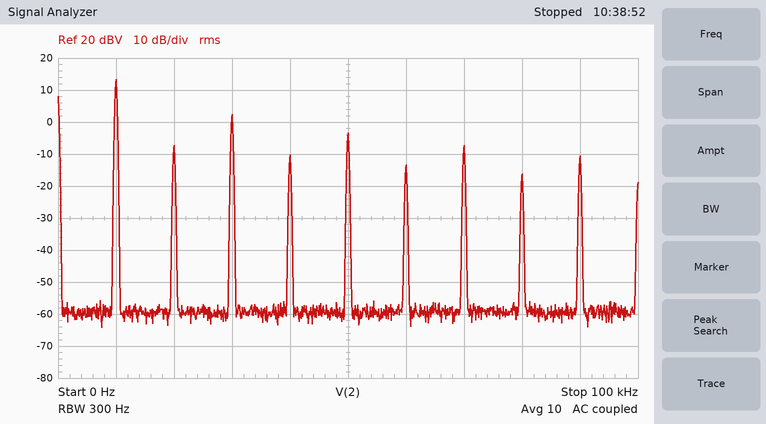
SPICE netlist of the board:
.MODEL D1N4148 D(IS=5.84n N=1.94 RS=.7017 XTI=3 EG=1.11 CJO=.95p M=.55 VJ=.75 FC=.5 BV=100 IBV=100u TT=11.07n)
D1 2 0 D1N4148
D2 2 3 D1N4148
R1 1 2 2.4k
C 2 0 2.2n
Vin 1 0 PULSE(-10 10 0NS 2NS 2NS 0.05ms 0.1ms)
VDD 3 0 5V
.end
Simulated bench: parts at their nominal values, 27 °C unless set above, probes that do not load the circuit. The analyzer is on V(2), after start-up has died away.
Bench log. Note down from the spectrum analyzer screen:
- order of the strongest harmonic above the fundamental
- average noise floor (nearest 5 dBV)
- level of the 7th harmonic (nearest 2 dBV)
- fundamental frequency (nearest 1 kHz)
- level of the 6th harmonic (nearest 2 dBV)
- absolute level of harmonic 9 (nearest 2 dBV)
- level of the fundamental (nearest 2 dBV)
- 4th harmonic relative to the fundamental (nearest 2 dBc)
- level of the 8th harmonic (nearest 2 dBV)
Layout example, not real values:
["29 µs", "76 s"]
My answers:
["3", "-60 dBV", "-8 dBV", "10 kHz", "-14 dBV", "-10 dBV", "14 dBV", "-24 dBc", "-16 dBV"]
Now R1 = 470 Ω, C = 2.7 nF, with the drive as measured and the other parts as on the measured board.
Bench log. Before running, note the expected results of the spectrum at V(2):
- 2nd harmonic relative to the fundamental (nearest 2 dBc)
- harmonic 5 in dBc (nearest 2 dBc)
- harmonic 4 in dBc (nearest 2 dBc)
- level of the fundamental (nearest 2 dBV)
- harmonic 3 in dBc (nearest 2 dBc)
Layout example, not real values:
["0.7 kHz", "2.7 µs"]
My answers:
["-32 dBc", "-14 dBc", "-32 dBc", "14 dBV", "-10 dBc"]
